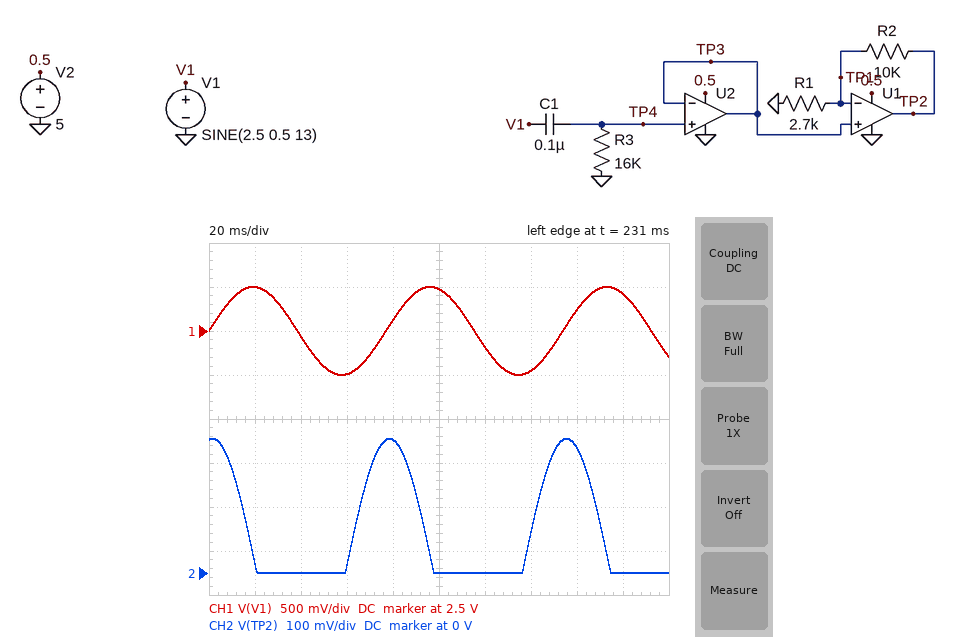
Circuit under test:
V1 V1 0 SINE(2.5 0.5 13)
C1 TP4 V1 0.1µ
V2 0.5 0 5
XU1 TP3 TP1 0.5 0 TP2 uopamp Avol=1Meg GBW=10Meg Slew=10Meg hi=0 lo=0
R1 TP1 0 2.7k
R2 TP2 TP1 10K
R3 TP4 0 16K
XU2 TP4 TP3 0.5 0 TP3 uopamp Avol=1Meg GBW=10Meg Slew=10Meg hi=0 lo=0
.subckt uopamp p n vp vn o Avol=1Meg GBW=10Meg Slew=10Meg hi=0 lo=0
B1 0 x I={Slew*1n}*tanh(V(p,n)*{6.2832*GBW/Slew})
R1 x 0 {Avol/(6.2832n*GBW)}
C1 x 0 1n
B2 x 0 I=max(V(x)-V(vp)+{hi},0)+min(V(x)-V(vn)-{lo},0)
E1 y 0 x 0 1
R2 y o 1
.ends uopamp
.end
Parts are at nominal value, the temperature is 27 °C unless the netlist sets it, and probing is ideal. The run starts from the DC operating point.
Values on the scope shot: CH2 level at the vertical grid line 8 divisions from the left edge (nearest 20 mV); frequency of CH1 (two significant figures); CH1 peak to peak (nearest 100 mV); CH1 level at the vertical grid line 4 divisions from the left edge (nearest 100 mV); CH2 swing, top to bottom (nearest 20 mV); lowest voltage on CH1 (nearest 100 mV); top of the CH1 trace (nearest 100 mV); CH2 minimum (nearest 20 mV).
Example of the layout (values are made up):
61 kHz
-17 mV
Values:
280 mV
13 Hz
1.0 V
2.6 V
300 mV
2.0 V
3.0 V
0 V
